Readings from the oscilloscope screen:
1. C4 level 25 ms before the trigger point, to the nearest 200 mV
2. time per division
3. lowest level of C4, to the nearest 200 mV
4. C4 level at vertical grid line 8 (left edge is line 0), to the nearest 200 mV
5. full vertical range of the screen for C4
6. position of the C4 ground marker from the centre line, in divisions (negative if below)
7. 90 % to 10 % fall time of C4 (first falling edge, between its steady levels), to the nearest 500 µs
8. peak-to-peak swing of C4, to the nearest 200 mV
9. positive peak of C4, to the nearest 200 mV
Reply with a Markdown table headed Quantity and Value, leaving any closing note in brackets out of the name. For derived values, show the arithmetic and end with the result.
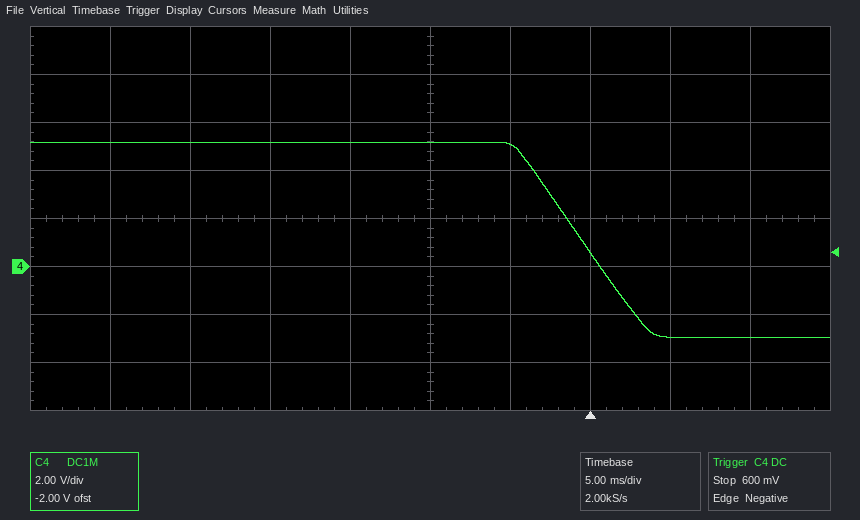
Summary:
| Quantity | Value |
|---|---|
| C4 level 25 ms before the trigger point, to the nearest 200 mV | 5.2 V |
| time per division | 5 ms |
| lowest level of C4, to the nearest 200 mV | -3.0 V |
| C4 level at vertical grid line 8 (left edge is line 0), to the nearest 200 mV | -3.0 V |
| full vertical range of the screen for C4 | 16 V |
| position of the C4 ground marker from the centre line, in divisions | -1.0 div |
| 90 % to 10 % fall time of C4 (first falling edge, between its steady levels), to the nearest 500 µs | 7.0 ms |
| peak-to-peak swing of C4, to the nearest 200 mV | 5.2 V − (-3.0 V) = 8.2 V |
| positive peak of C4, to the nearest 200 mV | 5.2 V |
